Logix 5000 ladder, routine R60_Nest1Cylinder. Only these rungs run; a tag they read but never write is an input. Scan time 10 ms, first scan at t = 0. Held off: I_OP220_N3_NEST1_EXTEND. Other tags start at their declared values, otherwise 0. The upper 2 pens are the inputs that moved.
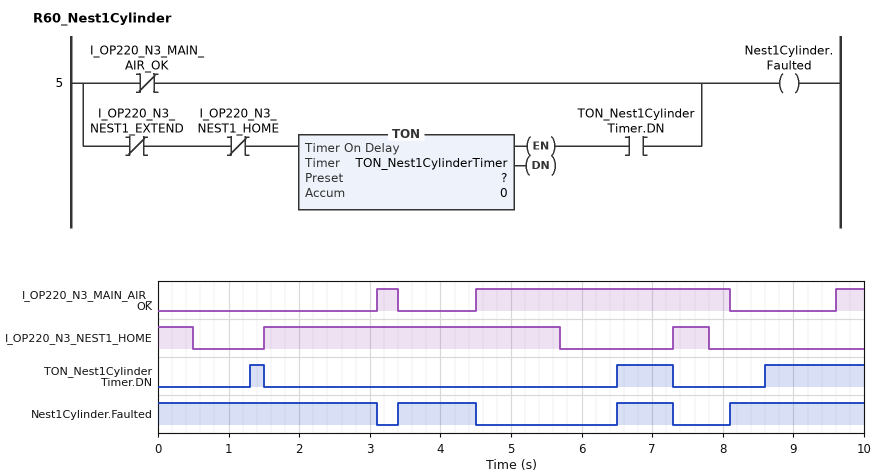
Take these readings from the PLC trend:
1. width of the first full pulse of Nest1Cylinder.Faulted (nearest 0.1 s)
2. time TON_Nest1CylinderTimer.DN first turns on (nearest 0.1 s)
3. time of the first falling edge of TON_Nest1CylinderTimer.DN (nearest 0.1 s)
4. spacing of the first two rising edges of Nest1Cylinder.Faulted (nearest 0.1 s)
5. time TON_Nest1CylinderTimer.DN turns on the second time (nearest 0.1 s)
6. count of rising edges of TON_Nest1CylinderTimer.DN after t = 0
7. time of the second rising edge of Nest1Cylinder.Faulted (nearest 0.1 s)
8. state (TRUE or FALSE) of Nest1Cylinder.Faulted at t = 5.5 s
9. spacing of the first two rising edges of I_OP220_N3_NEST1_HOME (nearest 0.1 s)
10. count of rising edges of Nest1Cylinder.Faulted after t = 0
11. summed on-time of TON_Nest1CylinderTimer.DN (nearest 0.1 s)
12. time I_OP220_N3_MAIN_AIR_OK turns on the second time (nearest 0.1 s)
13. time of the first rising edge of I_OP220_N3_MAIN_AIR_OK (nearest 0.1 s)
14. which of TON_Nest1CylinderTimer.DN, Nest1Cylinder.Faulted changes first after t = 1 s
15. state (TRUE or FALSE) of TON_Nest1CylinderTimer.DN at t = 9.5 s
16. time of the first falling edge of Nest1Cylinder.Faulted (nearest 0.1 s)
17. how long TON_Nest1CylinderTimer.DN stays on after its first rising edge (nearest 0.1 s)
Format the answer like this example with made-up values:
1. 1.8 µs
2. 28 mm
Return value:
1. 1.1 s
2. 1.3 s
3. 1.5 s
4. 3.1 s
5. 6.5 s
6. 3
7. 6.5 s
8. FALSE
9. 5.8 s
10. 3
11. 2.4 s
12. 4.5 s
13. 3.1 s
14. TON_Nest1CylinderTimer.DN
15. TRUE
16. 3.1 s
17. 0.2 s
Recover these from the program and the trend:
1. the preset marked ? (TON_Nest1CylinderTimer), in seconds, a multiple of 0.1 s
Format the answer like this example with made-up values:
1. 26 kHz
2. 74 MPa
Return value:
1. 0.8 s
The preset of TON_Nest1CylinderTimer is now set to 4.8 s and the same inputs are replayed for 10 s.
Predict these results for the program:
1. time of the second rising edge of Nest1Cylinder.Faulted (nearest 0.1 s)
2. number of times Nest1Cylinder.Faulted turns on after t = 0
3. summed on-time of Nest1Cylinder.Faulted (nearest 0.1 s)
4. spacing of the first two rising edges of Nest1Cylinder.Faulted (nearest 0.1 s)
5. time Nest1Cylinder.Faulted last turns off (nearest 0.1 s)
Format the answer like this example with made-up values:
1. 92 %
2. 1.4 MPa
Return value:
1. 8.1 s
2. 2
3. 5.7 s
4. 4.7 s
5. 9.6 s
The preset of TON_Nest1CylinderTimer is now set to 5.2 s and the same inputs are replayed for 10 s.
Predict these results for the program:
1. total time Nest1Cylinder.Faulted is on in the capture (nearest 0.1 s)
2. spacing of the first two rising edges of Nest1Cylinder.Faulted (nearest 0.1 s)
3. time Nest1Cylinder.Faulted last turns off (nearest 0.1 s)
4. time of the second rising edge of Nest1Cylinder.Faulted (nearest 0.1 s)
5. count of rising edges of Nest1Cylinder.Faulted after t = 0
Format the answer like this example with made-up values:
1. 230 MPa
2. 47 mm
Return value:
1. 5.7 s
2. 4.7 s
3. 9.6 s
4. 8.1 s
5. 2
